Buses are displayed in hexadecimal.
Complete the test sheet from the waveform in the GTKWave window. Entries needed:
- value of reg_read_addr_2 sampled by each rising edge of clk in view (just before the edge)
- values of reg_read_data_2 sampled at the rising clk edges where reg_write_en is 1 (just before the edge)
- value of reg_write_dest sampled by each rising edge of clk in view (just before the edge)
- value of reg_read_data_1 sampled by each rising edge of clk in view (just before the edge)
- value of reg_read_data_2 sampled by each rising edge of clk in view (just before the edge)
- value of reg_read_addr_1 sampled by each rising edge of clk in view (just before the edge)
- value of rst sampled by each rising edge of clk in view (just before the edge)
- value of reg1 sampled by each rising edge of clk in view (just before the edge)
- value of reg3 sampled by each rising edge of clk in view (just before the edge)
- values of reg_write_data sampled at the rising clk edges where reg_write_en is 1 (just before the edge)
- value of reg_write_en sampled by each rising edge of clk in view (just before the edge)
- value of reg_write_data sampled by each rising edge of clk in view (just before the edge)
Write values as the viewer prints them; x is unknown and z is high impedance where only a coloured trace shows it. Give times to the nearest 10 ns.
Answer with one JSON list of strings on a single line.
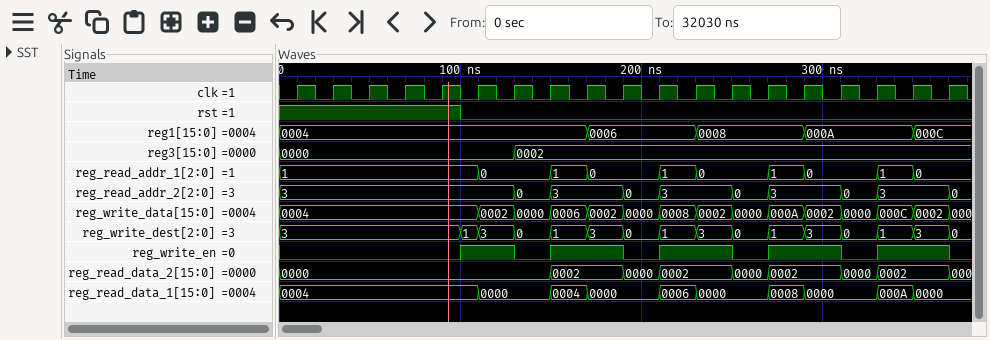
["3, 3, 3, 3, 3, 3, 3, 0, 3, 3, 0, 3, 3, 0, 3, 3, 0, 3, 3", "0000, 0000, 0002, 0002, 0002, 0002, 0002, 0002, 0002, 0002", "3, 3, 3, 3, 3, 1, 3, 0, 1, 3, 0, 1, 3, 0, 1, 3, 0, 1, 3", "0004, 0004, 0004, 0004, 0004, 0004, 0000, 0000, 0004, 0000, 0000, 0006, 0000, 0000, 0008, 0000, 0000, 000A, 0000", "0000, 0000, 0000, 0000, 0000, 0000, 0000, 0000, 0002, 0002, 0000, 0002, 0002, 0000, 0002, 0002, 0000, 0002, 0002", "1, 1, 1, 1, 1, 1, 0, 0, 1, 0, 0, 1, 0, 0, 1, 0, 0, 1, 0", "1 1 1 1 1 0 0 0 0 0 0 0 0 0 0 0 0 0 0", "0004, 0004, 0004, 0004, 0004, 0004, 0004, 0004, 0004, 0006, 0006, 0006, 0008, 0008, 0008, 000A, 000A, 000A, 000C", "0000, 0000, 0000, 0000, 0000, 0000, 0000, 0002, 0002, 0002, 0002, 0002, 0002, 0002, 0002, 0002, 0002, 0002, 0002", "0004, 0002, 0006, 0002, 0008, 0002, 000A, 0002, 000C, 0002", "0 0 0 0 0 1 1 0 1 1 0 1 1 0 1 1 0 1 1", "0004, 0004, 0004, 0004, 0004, 0004, 0002, 0000, 0006, 0002, 0000, 0008, 0002, 0000, 000A, 0002, 0000, 000C, 0002"]
